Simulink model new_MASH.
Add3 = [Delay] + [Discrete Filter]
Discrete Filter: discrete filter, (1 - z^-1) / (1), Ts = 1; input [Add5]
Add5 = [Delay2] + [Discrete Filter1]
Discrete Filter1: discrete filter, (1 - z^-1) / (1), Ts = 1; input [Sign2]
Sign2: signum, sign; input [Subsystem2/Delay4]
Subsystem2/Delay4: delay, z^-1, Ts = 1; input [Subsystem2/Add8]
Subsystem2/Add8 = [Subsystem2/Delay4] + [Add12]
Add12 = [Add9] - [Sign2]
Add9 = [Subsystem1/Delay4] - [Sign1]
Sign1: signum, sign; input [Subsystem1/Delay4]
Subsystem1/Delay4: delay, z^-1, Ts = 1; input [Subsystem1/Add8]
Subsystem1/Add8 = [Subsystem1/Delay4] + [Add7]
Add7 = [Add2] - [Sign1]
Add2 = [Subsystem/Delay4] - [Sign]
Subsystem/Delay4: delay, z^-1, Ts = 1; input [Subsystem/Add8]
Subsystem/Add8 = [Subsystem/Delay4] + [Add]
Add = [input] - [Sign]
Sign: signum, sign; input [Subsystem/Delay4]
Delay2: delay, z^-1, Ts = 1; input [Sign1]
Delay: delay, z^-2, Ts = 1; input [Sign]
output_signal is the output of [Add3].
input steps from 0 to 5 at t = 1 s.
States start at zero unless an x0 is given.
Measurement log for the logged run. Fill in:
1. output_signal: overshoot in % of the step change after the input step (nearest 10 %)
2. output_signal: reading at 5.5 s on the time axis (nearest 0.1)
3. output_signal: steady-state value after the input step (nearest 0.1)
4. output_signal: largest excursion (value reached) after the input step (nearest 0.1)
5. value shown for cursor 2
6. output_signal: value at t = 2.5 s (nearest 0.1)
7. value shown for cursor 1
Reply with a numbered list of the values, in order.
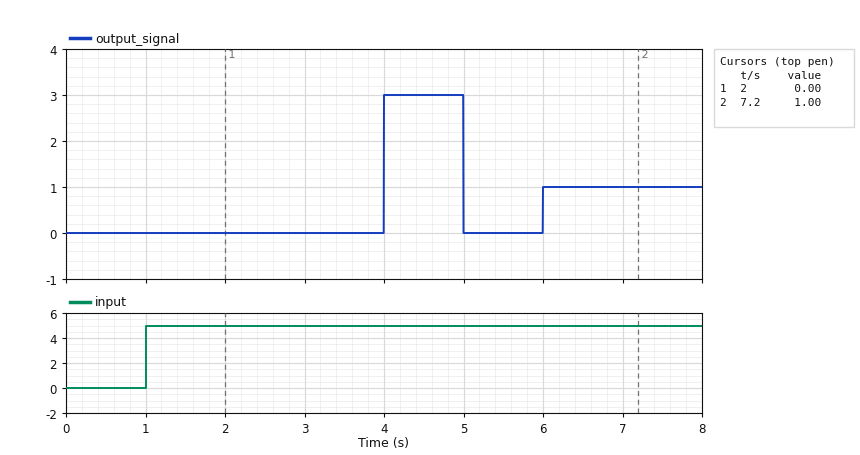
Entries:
1. 200 %
2. 0.0
3. 1.0
4. 3.0
5. 1.00
6. 0.0
7. 0.00
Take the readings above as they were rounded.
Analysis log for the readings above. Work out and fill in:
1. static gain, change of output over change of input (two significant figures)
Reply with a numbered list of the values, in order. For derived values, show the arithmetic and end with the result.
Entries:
1. (1 - 0) / (5 - 0) = 0.20
